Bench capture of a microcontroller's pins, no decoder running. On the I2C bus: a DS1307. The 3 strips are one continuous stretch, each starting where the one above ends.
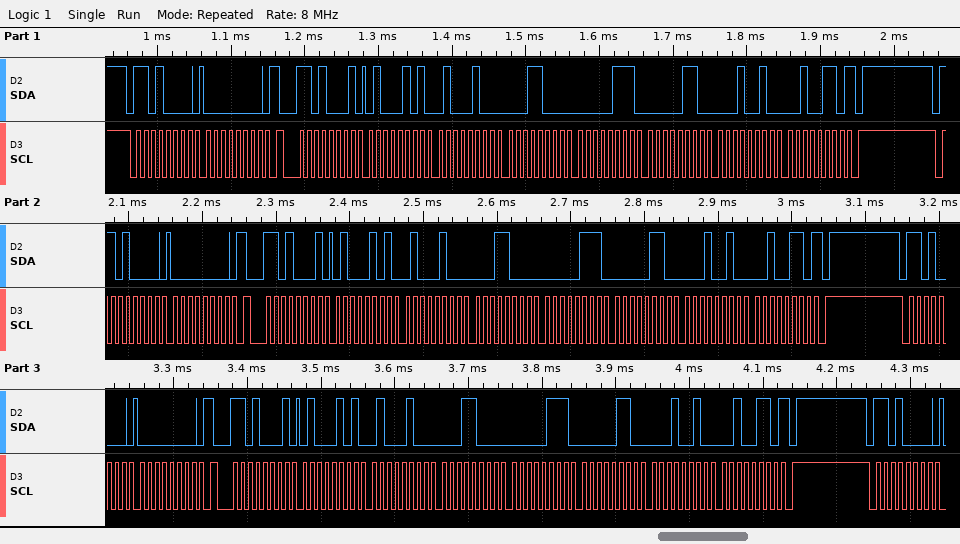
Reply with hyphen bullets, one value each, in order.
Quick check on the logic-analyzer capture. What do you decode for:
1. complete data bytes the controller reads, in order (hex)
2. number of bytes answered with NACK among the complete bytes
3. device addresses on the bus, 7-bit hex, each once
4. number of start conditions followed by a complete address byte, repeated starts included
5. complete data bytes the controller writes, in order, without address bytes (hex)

- 45 44 18 07 06 12 26 45 44 18 07 06 12 26 45 44 18 07 06 12 26
- 3
- 0x68
- 7
- 00 00 00
